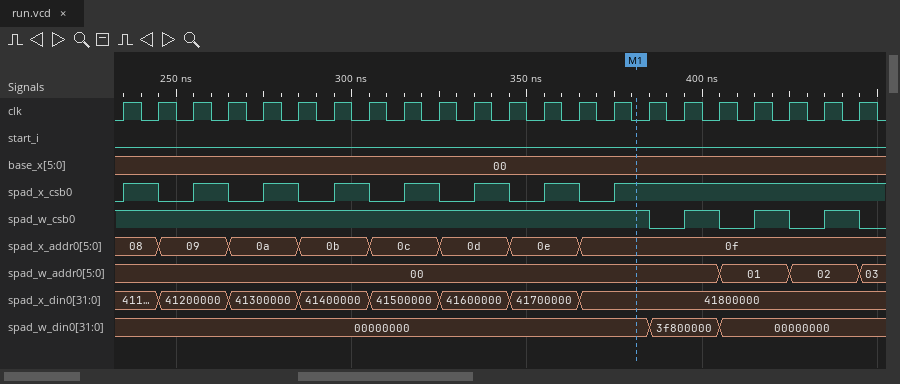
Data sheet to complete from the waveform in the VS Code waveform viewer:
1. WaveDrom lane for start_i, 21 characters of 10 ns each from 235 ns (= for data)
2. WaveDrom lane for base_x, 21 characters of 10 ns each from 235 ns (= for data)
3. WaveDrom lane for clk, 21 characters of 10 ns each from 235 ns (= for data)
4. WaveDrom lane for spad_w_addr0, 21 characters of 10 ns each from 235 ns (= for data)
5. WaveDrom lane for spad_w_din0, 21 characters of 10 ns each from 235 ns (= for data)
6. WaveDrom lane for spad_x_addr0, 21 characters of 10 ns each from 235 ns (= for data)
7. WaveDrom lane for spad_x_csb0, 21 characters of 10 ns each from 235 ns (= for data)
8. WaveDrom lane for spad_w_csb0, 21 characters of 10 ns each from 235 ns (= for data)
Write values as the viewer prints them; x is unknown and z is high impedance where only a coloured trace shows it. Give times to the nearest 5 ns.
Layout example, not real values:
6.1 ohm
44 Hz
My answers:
{name: 'start_i', wave: '0....................'}
{name: 'base_x', wave: '=....................', data: '00'}
{name: 'clk', wave: 'p....................'}
{name: 'spad_w_addr0', wave: '=................=.=.', data: '00 01 02'}
{name: 'spad_w_din0', wave: '=..............=.=...', data: '00000000 3f800000 00000000'}
{name: 'spad_x_addr0', wave: '==.=.=.=.=.=.=.......', data: '08 09 0a 0b 0c 0d 0e 0f'}
{name: 'spad_x_csb0', wave: '101010101010101......'}
{name: 'spad_w_csb0', wave: '1..............010101'}
